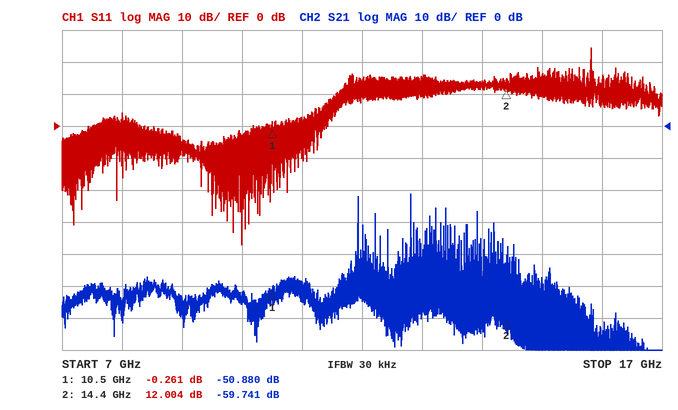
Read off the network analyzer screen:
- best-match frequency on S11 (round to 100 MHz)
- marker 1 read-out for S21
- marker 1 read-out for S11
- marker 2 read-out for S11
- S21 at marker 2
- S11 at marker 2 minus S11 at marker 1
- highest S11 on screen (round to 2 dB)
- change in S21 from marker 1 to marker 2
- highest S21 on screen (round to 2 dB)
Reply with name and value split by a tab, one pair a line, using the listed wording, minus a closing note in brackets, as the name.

best-match frequency on S11	10.0 GHz
marker 1 read-out for S21	-50.880 dB
marker 1 read-out for S11	-0.261 dB
marker 2 read-out for S11	12.004 dB
S21 at marker 2	-59.741 dB
S11 at marker 2 minus S11 at marker 1	12.265 dB
highest S11 on screen	24 dB
change in S21 from marker 1 to marker 2	-8.861 dB
highest S21 on screen	-22 dB
